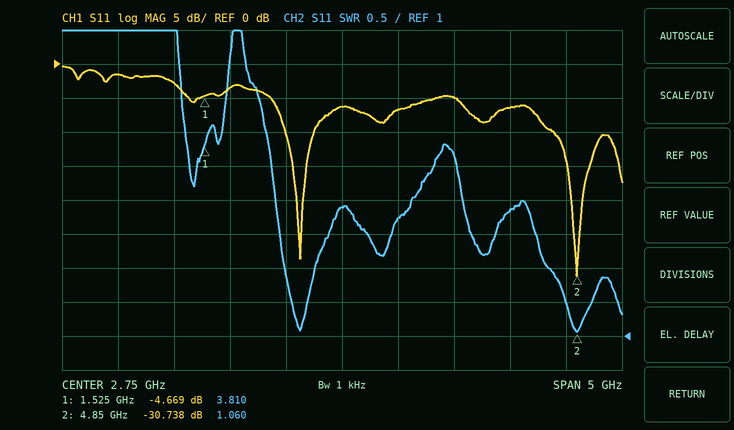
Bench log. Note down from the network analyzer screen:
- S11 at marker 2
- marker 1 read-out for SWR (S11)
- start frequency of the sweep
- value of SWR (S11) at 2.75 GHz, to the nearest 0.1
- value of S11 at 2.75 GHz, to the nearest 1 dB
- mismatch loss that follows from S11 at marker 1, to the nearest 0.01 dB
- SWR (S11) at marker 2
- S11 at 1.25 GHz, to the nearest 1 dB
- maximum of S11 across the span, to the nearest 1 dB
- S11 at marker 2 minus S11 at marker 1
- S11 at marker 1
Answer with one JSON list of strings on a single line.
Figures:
["-30.738 dB", "3.810", "250 MHz", "2.9", "-6 dB", "1.81 dB", "1.060", "-3 dB", "0 dB", "-26.069 dB", "-4.669 dB"]
